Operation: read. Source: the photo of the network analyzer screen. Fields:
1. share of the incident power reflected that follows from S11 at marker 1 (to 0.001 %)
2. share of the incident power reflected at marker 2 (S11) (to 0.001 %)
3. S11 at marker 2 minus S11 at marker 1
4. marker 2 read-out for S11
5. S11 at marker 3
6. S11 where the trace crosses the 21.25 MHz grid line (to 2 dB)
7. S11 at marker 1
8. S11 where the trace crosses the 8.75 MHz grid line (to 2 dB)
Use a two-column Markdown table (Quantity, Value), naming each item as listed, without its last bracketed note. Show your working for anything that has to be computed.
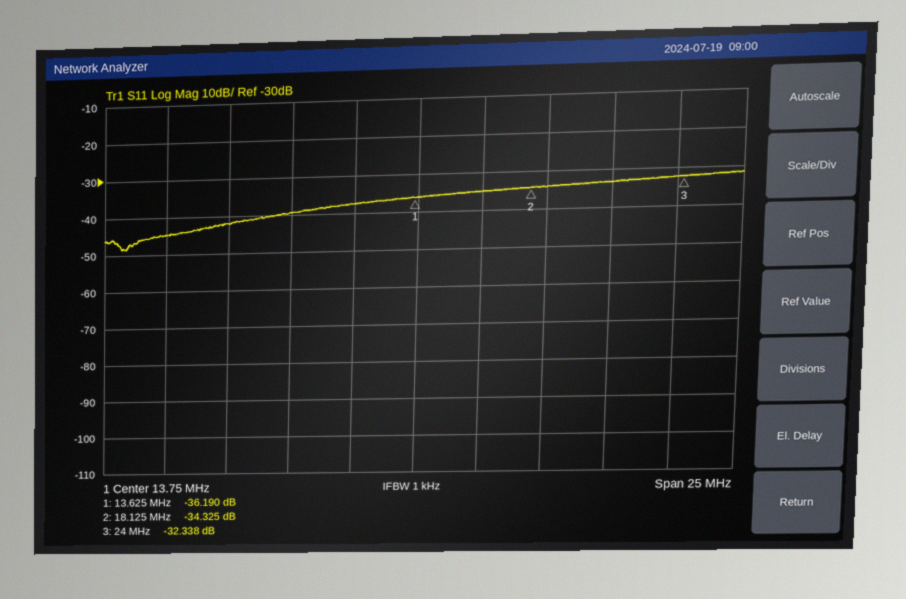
| Quantity | Value |
|---|---|
| share of the incident power reflected that follows from S11 at marker 1 | 10^(-36.19/10) ≈ 0.024 % |
| share of the incident power reflected at marker 2 (S11) | 10^(-34.325/10) ≈ 0.037 % |
| S11 at marker 2 minus S11 at marker 1 | -34.325 − (-36.19) = 1.865 dB |
| marker 2 read-out for S11 | -34.325 dB |
| S11 at marker 3 | -32.338 dB |
| S11 where the trace crosses the 21.25 MHz grid line | -34 dB |
| S11 at marker 1 | -36.190 dB |
| S11 where the trace crosses the 8.75 MHz grid line | -40 dB |
